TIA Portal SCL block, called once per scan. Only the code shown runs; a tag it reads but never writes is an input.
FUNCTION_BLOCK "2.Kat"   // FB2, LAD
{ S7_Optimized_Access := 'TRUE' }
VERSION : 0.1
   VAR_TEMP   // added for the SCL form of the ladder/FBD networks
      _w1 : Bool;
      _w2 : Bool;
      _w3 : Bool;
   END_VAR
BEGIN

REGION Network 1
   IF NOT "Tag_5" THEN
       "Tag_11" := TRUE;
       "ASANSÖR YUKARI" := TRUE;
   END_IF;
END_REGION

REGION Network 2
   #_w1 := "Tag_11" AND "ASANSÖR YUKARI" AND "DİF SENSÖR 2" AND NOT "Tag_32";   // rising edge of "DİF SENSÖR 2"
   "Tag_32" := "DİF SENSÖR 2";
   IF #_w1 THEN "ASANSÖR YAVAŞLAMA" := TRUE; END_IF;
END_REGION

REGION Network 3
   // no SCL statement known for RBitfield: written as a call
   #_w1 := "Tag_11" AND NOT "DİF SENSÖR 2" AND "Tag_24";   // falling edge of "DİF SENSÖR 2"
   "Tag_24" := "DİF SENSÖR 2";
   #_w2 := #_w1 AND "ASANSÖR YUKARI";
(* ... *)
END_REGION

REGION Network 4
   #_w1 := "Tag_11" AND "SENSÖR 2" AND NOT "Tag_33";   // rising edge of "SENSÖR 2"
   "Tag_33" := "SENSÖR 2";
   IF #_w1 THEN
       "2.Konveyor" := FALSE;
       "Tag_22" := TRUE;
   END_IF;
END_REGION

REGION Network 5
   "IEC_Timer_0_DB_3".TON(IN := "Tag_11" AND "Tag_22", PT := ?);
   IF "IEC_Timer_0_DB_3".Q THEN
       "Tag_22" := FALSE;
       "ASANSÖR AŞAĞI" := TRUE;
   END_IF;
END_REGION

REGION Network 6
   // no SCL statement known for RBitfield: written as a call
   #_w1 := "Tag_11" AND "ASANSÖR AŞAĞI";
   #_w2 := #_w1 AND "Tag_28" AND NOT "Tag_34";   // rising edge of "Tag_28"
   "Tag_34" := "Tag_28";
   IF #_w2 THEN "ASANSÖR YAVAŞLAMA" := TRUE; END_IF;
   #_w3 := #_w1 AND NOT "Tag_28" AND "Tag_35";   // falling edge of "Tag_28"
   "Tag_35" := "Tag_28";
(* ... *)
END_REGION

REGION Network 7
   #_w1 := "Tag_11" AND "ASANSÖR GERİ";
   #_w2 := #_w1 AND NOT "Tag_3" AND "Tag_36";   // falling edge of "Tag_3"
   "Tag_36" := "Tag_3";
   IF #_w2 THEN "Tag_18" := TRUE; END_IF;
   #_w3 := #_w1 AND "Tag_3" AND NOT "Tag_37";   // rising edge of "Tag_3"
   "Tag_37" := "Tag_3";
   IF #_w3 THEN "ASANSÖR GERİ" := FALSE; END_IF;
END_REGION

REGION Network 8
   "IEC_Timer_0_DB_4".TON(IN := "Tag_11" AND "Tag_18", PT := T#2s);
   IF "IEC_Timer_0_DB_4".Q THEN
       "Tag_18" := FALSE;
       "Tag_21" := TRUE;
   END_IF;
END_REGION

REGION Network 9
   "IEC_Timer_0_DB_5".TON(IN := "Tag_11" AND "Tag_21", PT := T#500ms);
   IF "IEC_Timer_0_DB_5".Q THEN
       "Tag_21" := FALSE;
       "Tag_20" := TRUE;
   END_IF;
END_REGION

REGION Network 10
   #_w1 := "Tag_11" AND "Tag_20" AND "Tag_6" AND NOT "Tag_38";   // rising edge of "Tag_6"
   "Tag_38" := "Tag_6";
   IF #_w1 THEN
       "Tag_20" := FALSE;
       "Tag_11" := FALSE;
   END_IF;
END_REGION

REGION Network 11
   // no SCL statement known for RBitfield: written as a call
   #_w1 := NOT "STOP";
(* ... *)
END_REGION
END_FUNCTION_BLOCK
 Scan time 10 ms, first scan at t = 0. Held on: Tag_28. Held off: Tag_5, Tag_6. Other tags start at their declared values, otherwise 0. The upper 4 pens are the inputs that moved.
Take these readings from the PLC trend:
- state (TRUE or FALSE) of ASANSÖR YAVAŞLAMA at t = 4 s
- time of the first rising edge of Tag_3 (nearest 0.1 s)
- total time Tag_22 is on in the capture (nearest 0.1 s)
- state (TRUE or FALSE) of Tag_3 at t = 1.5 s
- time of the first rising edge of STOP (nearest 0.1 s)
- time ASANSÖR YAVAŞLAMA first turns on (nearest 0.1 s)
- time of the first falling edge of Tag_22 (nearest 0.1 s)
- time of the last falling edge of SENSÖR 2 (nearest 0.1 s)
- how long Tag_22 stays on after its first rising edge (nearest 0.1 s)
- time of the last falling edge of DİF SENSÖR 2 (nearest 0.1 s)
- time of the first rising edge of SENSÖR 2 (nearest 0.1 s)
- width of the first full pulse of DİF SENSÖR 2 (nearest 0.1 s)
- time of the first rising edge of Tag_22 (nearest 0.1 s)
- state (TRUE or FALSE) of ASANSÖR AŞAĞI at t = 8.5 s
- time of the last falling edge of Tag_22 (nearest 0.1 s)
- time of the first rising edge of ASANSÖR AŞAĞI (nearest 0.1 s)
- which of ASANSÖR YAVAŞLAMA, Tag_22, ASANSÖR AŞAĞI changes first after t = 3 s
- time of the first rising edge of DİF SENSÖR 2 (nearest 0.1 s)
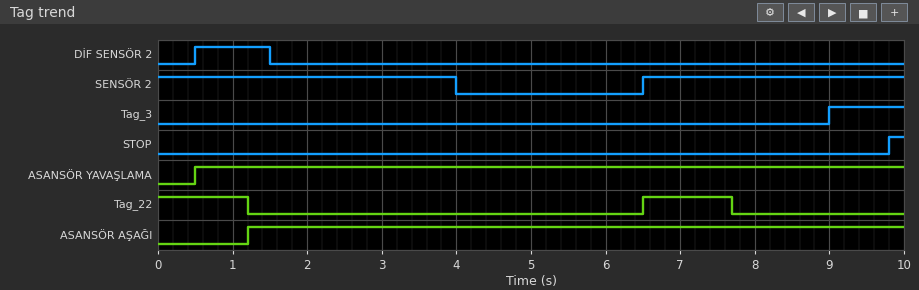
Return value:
TRUE
9.0 s
2.4 s
FALSE
9.8 s
0.5 s
1.2 s
4.0 s
1.2 s
1.5 s
6.5 s
1.0 s
6.5 s
TRUE
7.7 s
1.2 s
Tag_22
0.5 s
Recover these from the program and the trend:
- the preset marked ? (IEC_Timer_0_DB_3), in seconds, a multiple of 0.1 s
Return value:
1.2 s
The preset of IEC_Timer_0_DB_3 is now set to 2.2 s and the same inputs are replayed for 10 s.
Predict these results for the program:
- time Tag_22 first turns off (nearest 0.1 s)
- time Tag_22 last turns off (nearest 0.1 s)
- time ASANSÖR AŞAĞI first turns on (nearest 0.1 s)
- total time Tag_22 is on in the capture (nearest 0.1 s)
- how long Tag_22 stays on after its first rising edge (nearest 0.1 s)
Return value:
2.2 s
8.7 s
2.2 s
4.4 s
2.2 s
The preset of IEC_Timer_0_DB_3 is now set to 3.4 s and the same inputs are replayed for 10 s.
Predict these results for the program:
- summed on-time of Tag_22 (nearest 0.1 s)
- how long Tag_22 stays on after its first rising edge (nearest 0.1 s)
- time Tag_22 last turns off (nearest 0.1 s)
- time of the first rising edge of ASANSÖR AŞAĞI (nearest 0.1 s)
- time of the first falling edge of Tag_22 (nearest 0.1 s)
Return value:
6.8 s
3.4 s
9.9 s
3.4 s
3.4 s
